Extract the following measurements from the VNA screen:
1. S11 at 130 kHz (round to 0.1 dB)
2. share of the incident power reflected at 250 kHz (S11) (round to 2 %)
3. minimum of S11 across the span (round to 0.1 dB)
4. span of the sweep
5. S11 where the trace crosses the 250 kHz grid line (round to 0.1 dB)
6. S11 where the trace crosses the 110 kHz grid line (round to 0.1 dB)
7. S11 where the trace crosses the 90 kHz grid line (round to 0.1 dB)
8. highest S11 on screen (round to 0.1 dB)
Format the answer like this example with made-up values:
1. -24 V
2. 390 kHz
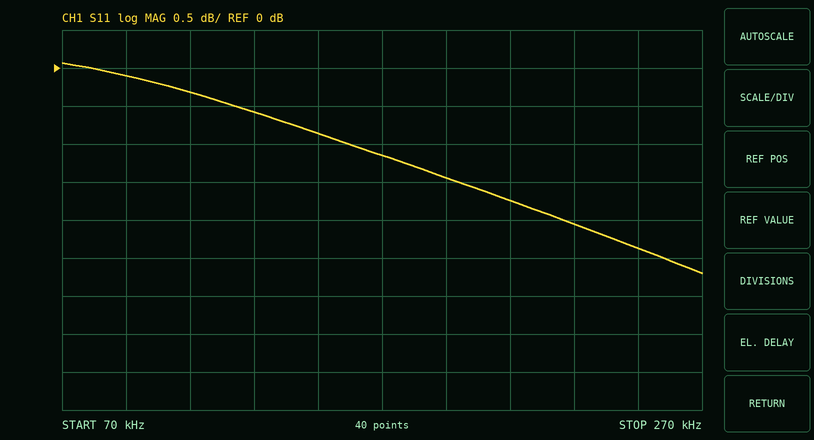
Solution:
1. -0.6 dB
2. 58 %
3. -2.7 dB
4. 200 kHz
5. -2.4 dB
6. -0.3 dB
7. -0.1 dB
8. 0.1 dB
